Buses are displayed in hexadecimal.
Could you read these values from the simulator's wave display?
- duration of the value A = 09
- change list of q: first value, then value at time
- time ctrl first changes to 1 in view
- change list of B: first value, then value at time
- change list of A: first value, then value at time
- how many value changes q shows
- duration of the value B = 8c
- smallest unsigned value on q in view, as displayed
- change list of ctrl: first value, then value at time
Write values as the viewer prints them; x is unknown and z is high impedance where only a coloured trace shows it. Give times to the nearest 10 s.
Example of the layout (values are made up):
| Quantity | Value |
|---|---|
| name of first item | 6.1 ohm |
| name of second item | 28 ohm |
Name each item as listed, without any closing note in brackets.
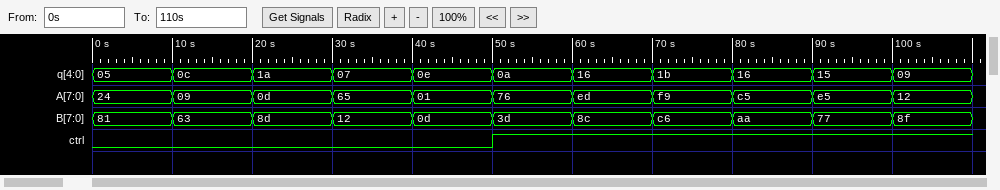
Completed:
| Quantity | Value |
|---|---|
| duration of the value A = 09 | 10 s |
| change list of q: first value, then value at time | 05, 0c at 10 s, 1a at 20 s, 07 at 30 s, 0e at 40 s, 0a at 50 s, 16 at 60 s, 1b at 70 s, 16 at 80 s, 15 at 90 s, 09 at 100 s |
| time ctrl first changes to 1 in view | 50 s |
| change list of B: first value, then value at time | 81, 63 at 10 s, 8d at 20 s, 12 at 30 s, 0d at 40 s, 3d at 50 s, 8c at 60 s, c6 at 70 s, aa at 80 s, 77 at 90 s, 8f at 100 s |
| change list of A: first value, then value at time | 24, 09 at 10 s, 0d at 20 s, 65 at 30 s, 01 at 40 s, 76 at 50 s, ed at 60 s, f9 at 70 s, c5 at 80 s, e5 at 90 s, 12 at 100 s |
| how many value changes q shows | 10 |
| duration of the value B = 8c | 10 s |
| smallest unsigned value on q in view, as displayed | 05 |
| change list of ctrl: first value, then value at time | 0, 1 at 50 s |
